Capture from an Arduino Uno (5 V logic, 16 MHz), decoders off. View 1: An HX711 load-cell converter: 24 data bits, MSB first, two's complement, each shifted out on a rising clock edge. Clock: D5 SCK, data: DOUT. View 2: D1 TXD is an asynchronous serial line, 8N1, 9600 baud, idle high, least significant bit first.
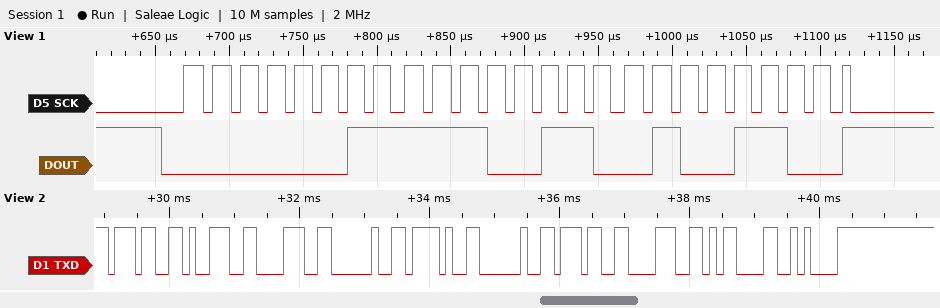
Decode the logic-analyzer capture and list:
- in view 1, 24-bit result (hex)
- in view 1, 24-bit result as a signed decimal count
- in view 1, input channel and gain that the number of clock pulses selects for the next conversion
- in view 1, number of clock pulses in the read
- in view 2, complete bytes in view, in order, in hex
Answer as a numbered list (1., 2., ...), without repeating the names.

1. 0x03E64C
2. 255564
3. channel A, gain 128
4. 25
5. 0x37 0x39 0x38 0x20 0x2F 0x20 0x37 0x38 0x0D 0x0A
